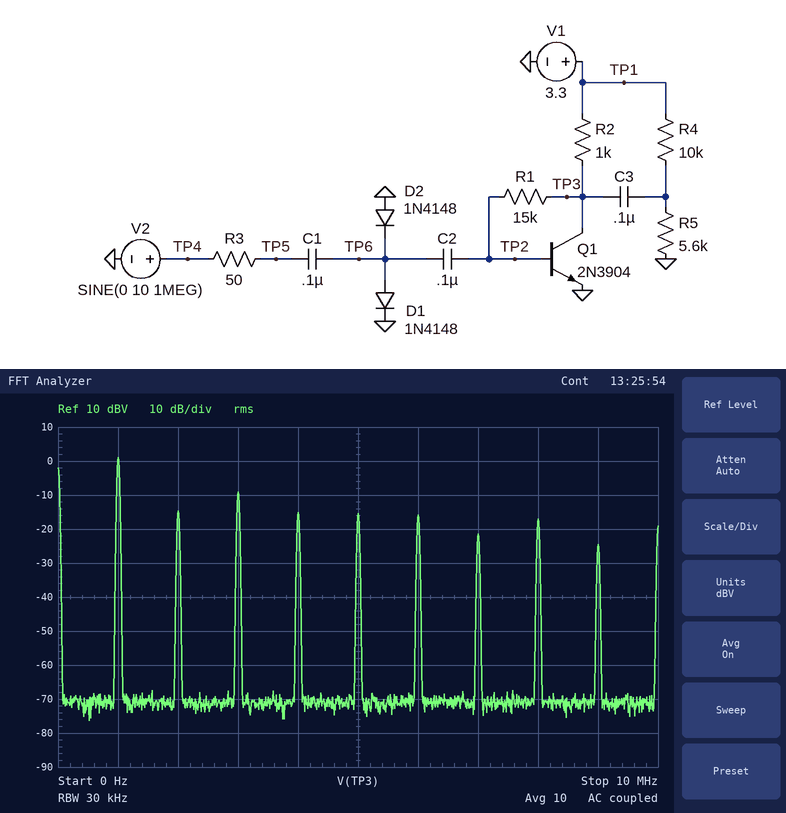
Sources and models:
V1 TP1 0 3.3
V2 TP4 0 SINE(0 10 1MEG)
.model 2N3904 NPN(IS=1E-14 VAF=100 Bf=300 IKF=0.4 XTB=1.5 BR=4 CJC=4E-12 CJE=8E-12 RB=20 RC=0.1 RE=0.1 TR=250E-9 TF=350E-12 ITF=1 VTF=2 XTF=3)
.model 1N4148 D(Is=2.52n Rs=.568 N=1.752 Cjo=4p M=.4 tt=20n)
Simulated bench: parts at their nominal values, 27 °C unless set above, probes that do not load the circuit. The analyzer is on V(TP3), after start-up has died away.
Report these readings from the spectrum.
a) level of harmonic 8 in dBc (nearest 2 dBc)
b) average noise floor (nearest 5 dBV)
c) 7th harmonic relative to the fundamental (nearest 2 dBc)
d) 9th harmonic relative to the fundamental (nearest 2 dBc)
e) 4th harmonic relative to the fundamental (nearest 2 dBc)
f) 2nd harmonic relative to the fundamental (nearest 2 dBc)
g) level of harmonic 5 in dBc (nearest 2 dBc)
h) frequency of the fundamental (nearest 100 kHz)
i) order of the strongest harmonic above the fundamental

-18 dBc
-70 dBV
-22 dBc
-26 dBc
-16 dBc
-16 dBc
-16 dBc
1.0 MHz
3
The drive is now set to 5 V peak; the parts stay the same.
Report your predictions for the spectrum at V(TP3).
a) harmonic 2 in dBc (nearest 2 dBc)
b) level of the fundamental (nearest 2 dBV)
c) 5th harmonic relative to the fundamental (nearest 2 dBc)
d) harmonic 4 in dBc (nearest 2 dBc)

-18 dBc
2 dBV
-16 dBc
-18 dBc
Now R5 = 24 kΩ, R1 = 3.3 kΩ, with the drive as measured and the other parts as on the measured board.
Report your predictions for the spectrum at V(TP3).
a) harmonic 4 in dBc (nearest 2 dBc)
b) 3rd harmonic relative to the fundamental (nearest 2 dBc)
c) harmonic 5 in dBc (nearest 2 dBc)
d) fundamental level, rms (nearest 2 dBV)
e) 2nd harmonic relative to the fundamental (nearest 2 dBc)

-12 dBc
-8 dBc
-12 dBc
0 dBV
-10 dBc
